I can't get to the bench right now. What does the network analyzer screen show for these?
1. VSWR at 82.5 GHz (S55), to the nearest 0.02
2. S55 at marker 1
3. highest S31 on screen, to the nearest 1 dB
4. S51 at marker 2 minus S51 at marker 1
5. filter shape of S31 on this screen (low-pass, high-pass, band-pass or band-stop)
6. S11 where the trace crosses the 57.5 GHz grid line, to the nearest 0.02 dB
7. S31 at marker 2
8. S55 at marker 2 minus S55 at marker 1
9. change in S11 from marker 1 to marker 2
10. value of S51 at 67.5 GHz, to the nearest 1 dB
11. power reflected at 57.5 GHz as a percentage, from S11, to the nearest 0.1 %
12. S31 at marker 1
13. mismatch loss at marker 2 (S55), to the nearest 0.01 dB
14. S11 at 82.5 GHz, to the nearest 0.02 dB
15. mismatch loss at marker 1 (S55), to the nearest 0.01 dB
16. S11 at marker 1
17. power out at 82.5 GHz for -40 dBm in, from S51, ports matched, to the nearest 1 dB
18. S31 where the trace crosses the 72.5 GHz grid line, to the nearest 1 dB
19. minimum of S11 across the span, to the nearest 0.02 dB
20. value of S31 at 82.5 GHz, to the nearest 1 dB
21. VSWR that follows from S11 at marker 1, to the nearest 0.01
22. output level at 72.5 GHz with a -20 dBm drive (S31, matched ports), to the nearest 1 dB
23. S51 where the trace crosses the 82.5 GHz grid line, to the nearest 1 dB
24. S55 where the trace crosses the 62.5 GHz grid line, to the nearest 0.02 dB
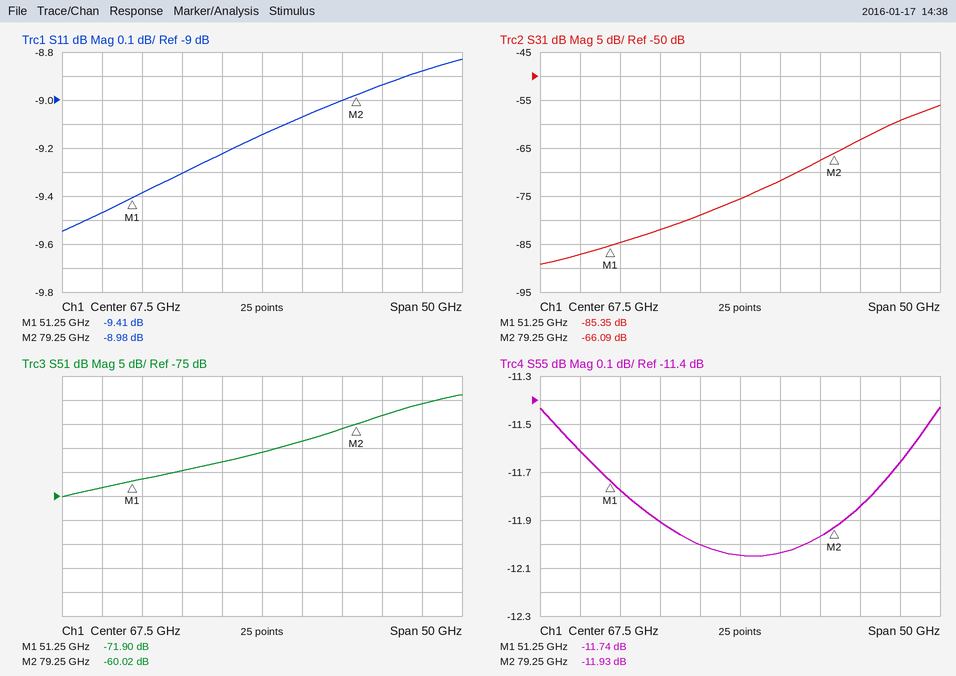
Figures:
1.68
-11.74 dB
-56 dB
11.88 dB
high-pass
-9.30 dB
-66.09 dB
-0.19 dB
0.43 dB
-66 dB
11.7 %
-85.35 dB
0.29 dB
-8.94 dB
0.30 dB
-9.41 dB
-98 dBm
-72 dB
-9.54 dB
-63 dB
2.02
-92 dBm
-58 dB
-12.00 dB
